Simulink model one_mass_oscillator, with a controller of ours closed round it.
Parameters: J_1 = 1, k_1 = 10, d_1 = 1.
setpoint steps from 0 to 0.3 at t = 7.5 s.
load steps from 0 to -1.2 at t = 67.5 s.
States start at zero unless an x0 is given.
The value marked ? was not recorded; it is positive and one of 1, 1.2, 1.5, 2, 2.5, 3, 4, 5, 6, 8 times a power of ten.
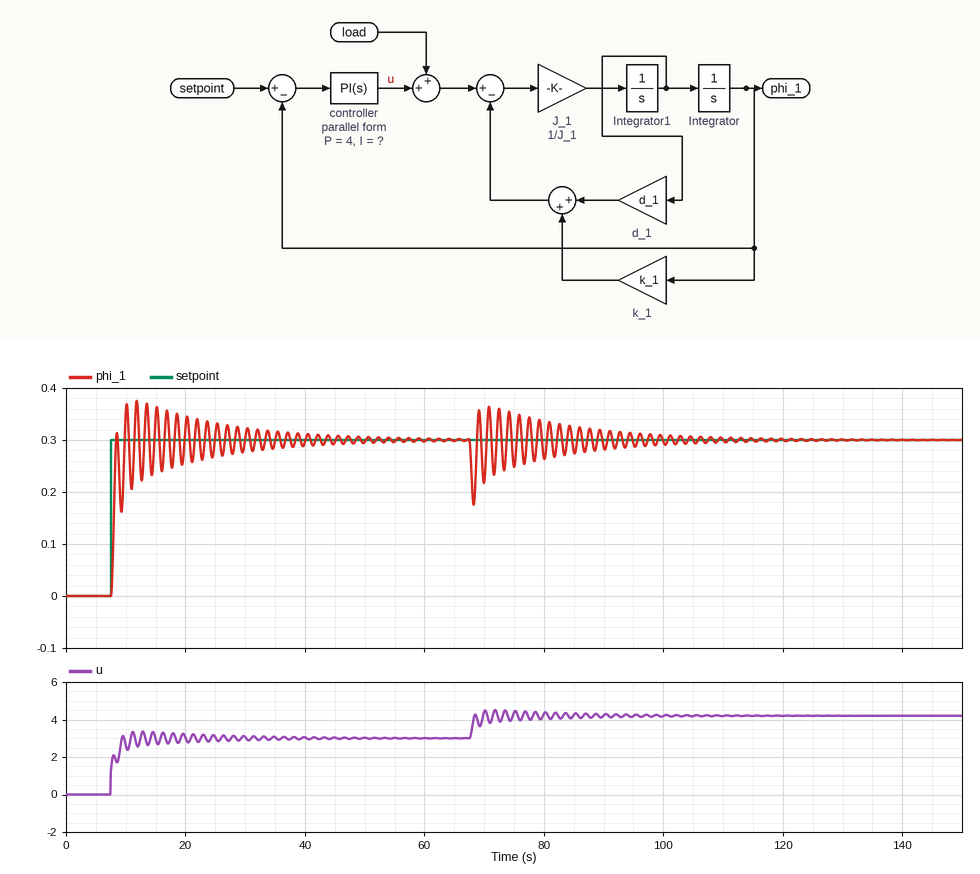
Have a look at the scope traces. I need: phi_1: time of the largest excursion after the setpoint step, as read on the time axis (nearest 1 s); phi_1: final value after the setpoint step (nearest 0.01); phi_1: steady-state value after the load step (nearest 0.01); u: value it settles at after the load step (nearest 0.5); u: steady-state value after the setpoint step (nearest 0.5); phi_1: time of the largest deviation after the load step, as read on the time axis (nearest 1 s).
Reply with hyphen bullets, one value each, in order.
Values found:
- 12 s
- 0.30
- 0.30
- 4.0
- 3.0
- 68 s
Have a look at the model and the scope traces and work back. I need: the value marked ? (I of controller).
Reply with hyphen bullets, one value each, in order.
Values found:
- 12
